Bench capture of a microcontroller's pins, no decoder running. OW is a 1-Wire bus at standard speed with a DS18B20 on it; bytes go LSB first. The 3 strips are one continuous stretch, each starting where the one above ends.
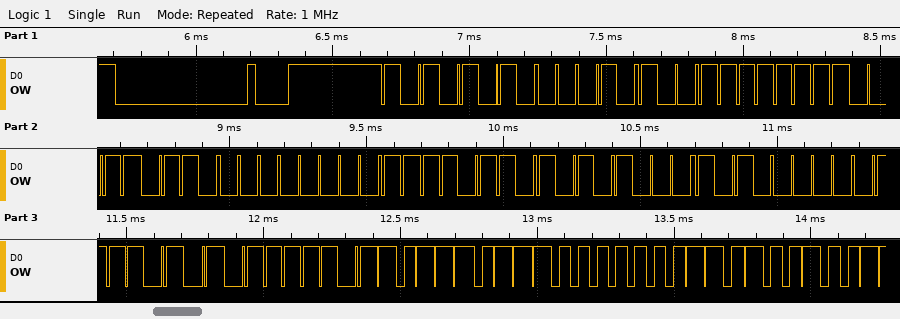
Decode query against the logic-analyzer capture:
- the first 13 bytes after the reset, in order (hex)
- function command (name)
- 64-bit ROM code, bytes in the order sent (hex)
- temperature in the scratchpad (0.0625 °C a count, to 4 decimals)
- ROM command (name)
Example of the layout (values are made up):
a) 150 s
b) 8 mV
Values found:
a) 55 28 FF 6C 00 6F 15 05 AE BE DD 01 4B
b) Read Scratchpad
c) 28 FF 6C 00 6F 15 05 AE
d) 29.8125 °C
e) Match ROM
